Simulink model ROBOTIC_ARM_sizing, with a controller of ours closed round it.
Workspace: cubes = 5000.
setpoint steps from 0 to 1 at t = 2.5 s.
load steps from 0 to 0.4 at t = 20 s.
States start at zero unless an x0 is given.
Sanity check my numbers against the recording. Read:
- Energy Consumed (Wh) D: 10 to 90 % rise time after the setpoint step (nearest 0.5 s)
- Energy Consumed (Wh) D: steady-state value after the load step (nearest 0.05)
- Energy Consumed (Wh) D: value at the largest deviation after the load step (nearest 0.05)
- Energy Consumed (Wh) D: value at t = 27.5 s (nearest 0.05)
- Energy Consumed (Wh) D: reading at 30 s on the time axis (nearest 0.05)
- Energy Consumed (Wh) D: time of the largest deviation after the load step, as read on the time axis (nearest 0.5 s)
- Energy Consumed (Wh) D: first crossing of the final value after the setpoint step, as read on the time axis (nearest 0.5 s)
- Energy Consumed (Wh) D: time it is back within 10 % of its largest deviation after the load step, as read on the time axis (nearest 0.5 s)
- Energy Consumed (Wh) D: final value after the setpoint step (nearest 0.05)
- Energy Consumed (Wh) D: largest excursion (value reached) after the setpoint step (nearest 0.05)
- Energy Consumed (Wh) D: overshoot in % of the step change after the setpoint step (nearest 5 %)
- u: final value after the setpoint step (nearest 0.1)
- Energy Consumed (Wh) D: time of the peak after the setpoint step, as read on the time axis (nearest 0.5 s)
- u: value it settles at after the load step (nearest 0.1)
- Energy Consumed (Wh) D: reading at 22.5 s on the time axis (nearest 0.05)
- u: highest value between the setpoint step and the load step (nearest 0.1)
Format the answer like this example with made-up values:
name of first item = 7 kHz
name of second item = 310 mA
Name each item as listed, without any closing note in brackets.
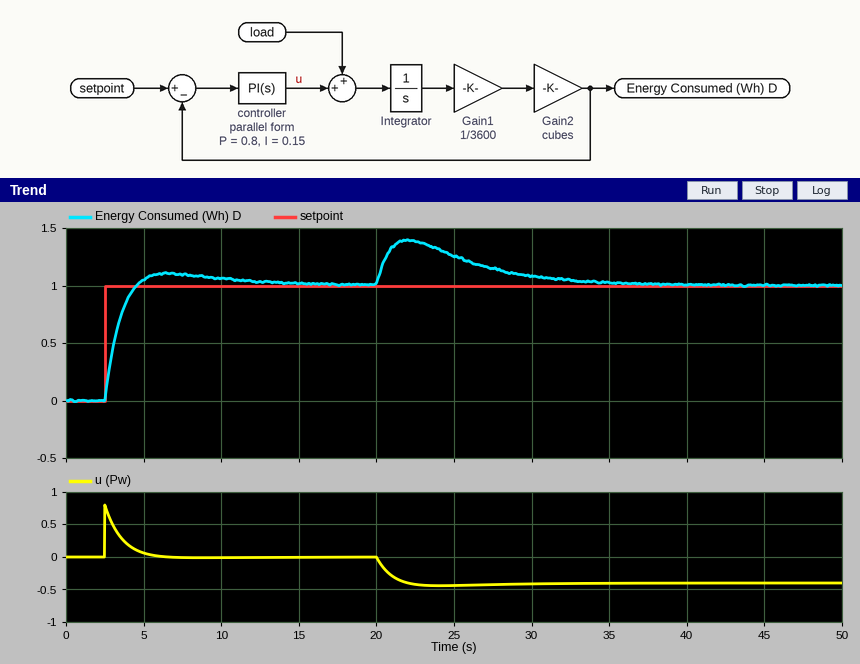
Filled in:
Energy Consumed (Wh) D: 10 to 90 % rise time after the setpoint step = 1.5 s
Energy Consumed (Wh) D: steady-state value after the load step = 1.00
Energy Consumed (Wh) D: value at the largest deviation after the load step = 1.40
Energy Consumed (Wh) D: value at t = 27.5 s = 1.15
Energy Consumed (Wh) D: reading at 30 s on the time axis = 1.10
Energy Consumed (Wh) D: time of the largest deviation after the load step, as read on the time axis = 22.0 s
Energy Consumed (Wh) D: first crossing of the final value after the setpoint step, as read on the time axis = 4.5 s
Energy Consumed (Wh) D: time it is back within 10 % of its largest deviation after the load step, as read on the time axis = 33.0 s
Energy Consumed (Wh) D: final value after the setpoint step = 1.00
Energy Consumed (Wh) D: largest excursion (value reached) after the setpoint step = 1.10
Energy Consumed (Wh) D: overshoot in % of the step change after the setpoint step = 10 %
u: final value after the setpoint step = 0.0
Energy Consumed (Wh) D: time of the peak after the setpoint step, as read on the time axis = 6.5 s
u: value it settles at after the load step = -0.4
Energy Consumed (Wh) D: reading at 22.5 s on the time axis = 1.40
u: highest value between the setpoint step and the load step = 0.8
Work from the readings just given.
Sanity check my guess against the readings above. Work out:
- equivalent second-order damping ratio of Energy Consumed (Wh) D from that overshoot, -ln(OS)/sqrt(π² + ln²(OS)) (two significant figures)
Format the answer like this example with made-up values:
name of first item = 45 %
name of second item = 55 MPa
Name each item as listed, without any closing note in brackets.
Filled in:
equivalent second-order damping ratio of Energy Consumed (Wh) D from that overshoot, -ln(OS)/sqrt(π² + ln²(OS)) = 0.59
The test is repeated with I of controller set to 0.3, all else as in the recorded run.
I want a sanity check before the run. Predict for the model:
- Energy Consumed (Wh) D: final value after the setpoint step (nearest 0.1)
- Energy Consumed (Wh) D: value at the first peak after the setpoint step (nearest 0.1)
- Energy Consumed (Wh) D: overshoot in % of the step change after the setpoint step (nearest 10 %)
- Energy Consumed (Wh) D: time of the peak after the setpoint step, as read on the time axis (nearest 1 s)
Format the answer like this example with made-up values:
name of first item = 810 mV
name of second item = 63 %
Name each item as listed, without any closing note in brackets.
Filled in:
Energy Consumed (Wh) D: final value after the setpoint step = 1.0
Energy Consumed (Wh) D: value at the first peak after the setpoint step = 1.2
Energy Consumed (Wh) D: overshoot in % of the step change after the setpoint step = 20 %
Energy Consumed (Wh) D: time of the peak after the setpoint step, as read on the time axis = 6 s
